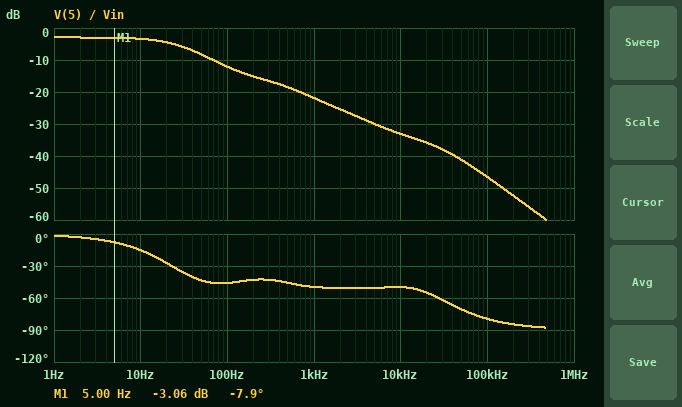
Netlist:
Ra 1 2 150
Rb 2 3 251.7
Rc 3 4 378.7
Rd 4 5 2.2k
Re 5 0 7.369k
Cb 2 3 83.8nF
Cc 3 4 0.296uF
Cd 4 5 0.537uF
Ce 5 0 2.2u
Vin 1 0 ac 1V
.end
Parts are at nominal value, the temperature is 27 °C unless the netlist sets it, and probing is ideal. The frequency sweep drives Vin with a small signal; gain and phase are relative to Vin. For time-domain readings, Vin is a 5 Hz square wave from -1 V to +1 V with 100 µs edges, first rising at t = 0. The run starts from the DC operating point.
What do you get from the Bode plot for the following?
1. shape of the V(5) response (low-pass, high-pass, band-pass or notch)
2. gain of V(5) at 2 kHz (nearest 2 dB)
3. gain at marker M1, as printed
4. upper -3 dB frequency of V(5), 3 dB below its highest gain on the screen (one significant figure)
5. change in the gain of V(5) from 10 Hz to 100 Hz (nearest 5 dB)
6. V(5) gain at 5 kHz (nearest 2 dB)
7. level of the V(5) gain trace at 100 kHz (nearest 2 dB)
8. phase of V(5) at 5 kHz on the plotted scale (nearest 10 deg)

low-pass
-26 dB
-3.06 dB
30 Hz
-10 dB
-30 dB
-46 dB
-50 deg
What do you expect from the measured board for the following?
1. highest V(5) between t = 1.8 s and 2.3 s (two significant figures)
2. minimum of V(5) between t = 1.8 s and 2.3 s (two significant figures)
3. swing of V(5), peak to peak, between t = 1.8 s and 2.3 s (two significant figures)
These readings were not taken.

710 mV
-710 mV
1.4 V
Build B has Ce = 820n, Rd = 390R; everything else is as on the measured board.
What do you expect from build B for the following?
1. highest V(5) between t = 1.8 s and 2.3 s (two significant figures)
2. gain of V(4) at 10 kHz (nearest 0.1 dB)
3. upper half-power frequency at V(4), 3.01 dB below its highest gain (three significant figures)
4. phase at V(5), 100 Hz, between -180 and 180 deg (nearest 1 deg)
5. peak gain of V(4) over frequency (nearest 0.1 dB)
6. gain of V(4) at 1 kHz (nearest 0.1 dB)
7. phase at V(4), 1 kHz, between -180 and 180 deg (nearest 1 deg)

860 mV
-16.7 dB
248 Hz
-26 deg
-0.8 dB
-7.7 dB
-32 deg
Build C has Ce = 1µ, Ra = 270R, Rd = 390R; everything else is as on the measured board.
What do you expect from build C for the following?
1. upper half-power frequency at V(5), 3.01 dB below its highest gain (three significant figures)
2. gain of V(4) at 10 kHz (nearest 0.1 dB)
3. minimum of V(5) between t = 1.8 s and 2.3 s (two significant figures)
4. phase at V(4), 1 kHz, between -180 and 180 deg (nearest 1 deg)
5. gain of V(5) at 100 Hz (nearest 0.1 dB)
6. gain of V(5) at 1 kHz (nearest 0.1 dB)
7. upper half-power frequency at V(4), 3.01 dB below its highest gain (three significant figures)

136 Hz
-19.5 dB
-850 mV
-36 deg
-3.3 dB
-16.6 dB
176 Hz
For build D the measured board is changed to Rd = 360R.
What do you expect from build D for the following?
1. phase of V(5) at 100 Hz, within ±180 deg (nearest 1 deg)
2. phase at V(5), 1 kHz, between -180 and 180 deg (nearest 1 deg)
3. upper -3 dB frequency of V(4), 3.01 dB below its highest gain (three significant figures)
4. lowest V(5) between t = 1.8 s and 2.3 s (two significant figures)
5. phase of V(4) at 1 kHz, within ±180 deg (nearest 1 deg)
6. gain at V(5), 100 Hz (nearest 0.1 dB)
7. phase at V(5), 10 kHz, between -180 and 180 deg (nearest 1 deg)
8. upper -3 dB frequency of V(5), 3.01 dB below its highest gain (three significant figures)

-51 deg
-59 deg
86.3 Hz
-870 mV
-30 deg
-6.0 dB
-50 deg
70.6 Hz
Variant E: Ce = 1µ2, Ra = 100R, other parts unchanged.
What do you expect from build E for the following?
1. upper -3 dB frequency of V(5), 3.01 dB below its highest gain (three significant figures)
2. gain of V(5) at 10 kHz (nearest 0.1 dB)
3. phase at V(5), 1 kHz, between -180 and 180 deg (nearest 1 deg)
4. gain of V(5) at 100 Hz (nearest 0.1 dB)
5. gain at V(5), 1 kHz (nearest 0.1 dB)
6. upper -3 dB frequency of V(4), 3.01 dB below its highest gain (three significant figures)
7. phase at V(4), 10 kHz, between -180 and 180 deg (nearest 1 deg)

57.1 Hz
-26.9 dB
-44 deg
-8.2 dB
-16.7 dB
493 Hz
-42 deg
